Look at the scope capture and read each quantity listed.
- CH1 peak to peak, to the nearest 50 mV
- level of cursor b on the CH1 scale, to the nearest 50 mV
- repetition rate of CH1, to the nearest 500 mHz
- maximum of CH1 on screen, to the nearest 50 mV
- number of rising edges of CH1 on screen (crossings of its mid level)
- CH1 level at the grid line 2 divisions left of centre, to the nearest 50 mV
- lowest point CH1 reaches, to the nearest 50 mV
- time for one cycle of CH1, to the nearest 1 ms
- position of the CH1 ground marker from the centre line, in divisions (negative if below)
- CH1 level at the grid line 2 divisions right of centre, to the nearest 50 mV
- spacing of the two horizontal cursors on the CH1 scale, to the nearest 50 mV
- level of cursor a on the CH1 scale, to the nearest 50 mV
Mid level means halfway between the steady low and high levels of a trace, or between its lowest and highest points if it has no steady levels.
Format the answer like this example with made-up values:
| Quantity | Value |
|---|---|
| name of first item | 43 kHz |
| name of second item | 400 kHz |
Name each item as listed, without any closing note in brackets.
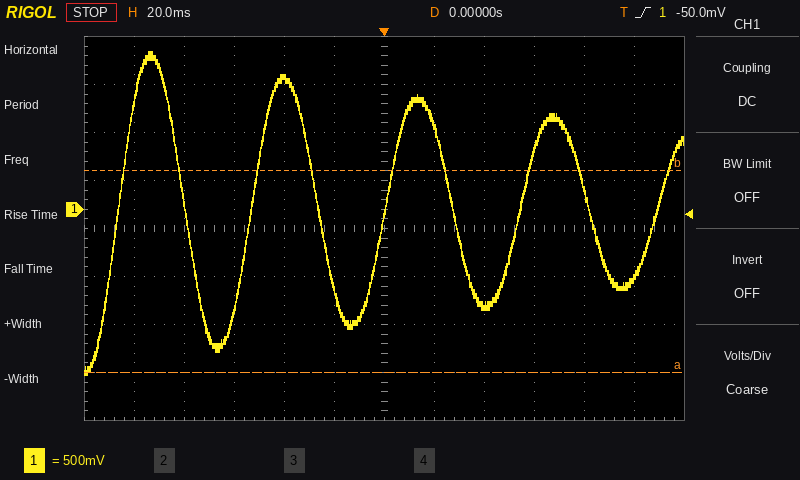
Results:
| Quantity | Value |
|---|---|
| CH1 peak to peak, to the nearest 50 mV | 3.35 V |
| level of cursor b on the CH1 scale, to the nearest 50 mV | 400 mV |
| repetition rate of CH1, to the nearest 500 mHz | 18.5 Hz |
| maximum of CH1 on screen, to the nearest 50 mV | 1.65 V |
| number of rising edges of CH1 on screen | 5 |
| CH1 level at the grid line 2 divisions left of centre, to the nearest 50 mV | 1.35 V |
| lowest point CH1 reaches, to the nearest 50 mV | -1.70 V |
| time for one cycle of CH1, to the nearest 1 ms | 54 ms |
| position of the CH1 ground marker from the centre line, in divisions | +0.4 div |
| CH1 level at the grid line 2 divisions right of centre, to the nearest 50 mV | -1.00 V |
| spacing of the two horizontal cursors on the CH1 scale, to the nearest 50 mV | 2.10 V |
| level of cursor a on the CH1 scale, to the nearest 50 mV | -1.70 V |
